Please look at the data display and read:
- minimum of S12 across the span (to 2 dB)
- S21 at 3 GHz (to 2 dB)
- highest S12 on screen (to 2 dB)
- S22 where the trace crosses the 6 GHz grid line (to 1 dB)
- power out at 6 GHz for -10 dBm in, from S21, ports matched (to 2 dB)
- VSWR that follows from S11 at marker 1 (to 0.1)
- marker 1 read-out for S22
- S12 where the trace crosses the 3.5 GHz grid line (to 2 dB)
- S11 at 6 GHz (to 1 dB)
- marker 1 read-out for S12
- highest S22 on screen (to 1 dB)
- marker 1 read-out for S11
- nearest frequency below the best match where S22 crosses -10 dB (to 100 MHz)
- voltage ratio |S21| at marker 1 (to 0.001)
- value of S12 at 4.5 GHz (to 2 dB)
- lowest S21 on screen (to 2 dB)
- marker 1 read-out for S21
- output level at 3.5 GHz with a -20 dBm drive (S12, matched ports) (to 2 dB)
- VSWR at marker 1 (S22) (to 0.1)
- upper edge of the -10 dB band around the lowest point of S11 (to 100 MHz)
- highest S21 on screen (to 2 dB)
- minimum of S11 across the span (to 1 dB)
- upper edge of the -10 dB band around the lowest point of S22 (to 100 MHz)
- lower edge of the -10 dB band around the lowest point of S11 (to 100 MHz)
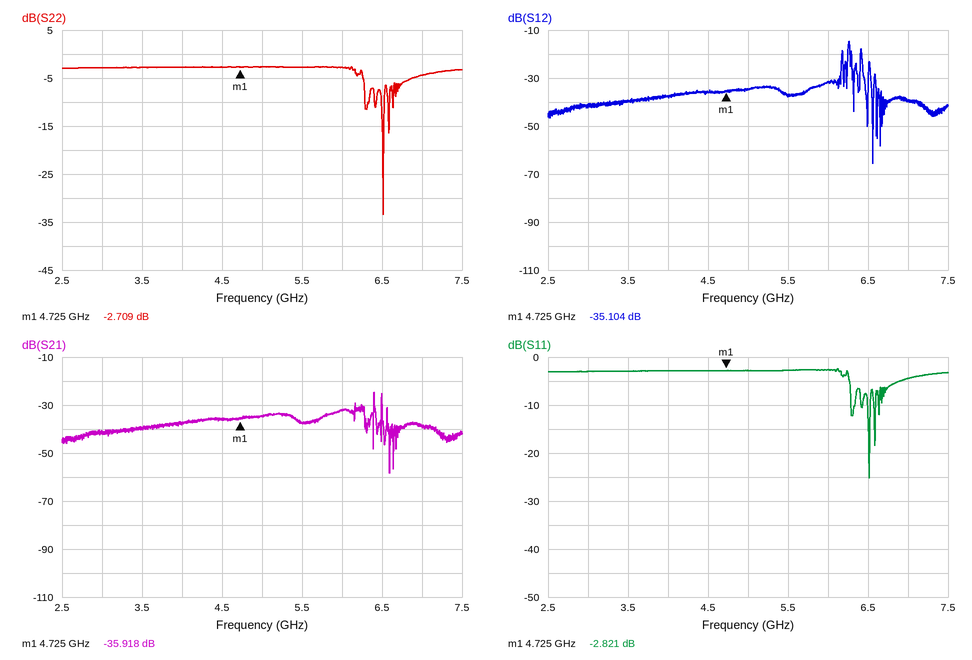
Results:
-66 dB
-42 dB
-14 dB
-3 dB
-42 dBm
6.2
-2.709 dB
-40 dB
-3 dB
-35.104 dB
-3 dB
-2.821 dB
6.5 GHz
0.016
-36 dB
-58 dB
-35.918 dB
-60 dBm
6.5
6.5 GHz
-24 dB
-25 dB
6.5 GHz
6.5 GHz
